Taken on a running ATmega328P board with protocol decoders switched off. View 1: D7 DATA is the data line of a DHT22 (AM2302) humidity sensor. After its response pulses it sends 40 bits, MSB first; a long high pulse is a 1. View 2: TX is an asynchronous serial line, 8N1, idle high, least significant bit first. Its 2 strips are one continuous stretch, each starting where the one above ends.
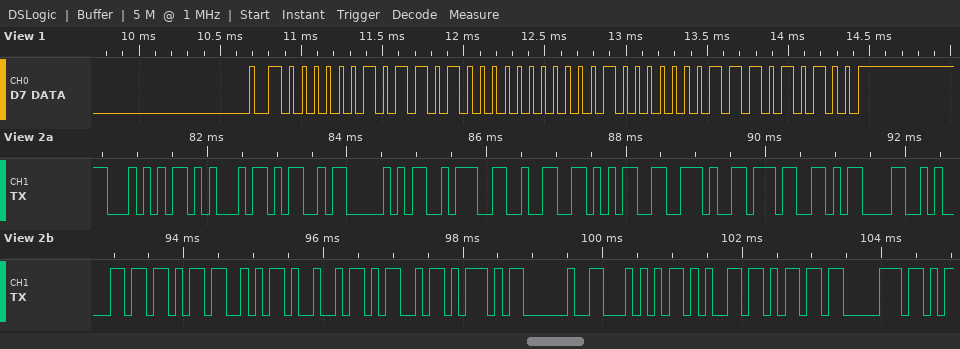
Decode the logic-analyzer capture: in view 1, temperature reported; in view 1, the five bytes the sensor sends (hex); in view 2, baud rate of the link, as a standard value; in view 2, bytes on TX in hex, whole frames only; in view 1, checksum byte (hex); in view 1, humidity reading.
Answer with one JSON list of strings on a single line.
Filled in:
["25.7 °C", "02 D0 01 01 D4", "9600 baud", "54 45 4D 50 3A 32 35 2E 37 0D 0A 5B 53 49 4D 5D 20 54 65 6D 70", "0xD4", "72.0 %"]
